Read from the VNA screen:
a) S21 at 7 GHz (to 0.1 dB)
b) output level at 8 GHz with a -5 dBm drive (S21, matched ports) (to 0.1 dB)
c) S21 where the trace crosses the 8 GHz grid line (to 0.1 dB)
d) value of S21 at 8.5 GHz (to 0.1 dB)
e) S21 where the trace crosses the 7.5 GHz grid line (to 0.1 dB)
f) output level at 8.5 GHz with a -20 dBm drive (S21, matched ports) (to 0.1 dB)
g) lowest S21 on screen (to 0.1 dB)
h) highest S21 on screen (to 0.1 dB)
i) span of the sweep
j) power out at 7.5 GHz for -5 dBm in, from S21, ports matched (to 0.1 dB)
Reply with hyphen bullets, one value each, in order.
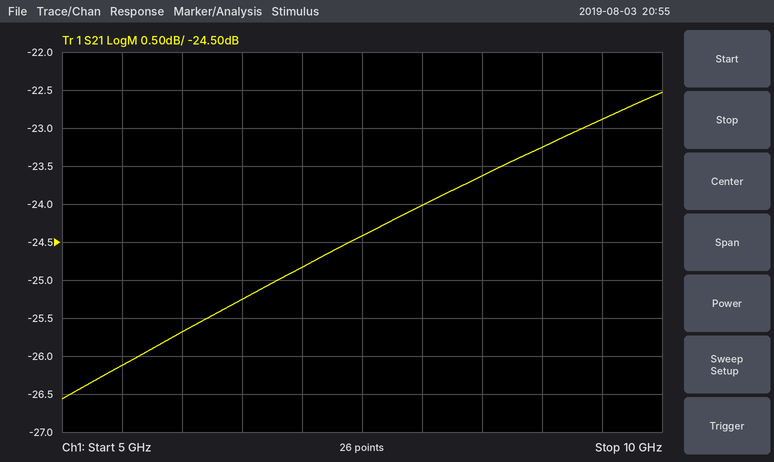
- -24.8 dB
- -29.0 dBm
- -24.0 dB
- -23.6 dB
- -24.4 dB
- -43.6 dBm
- -26.6 dB
- -22.5 dB
- 5 GHz
- -29.4 dBm
